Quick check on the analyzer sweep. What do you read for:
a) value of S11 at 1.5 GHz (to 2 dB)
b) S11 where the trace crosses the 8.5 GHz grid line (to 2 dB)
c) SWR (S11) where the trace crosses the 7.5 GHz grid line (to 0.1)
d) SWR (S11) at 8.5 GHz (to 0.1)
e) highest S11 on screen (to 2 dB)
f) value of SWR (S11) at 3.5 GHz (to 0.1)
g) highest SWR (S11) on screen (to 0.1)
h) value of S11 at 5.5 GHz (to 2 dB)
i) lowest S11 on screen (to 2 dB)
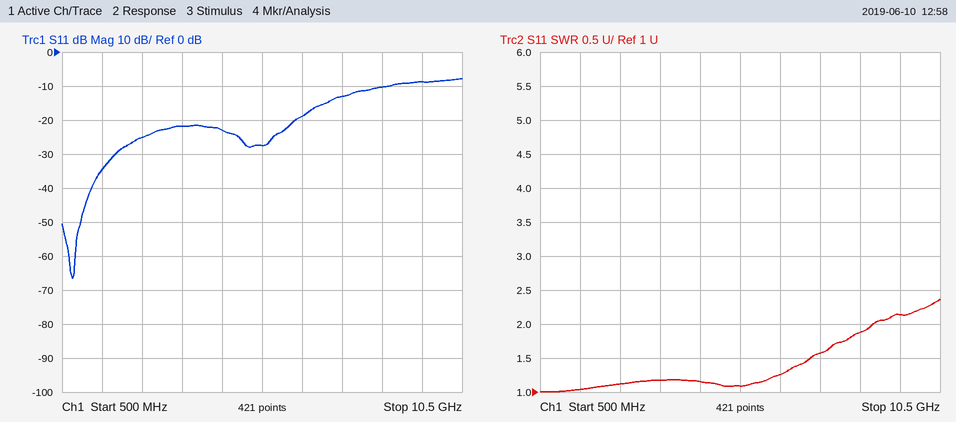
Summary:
-34 dB
-10 dB
1.6
1.9
-8 dB
1.2
2.4
-28 dB
-66 dB
